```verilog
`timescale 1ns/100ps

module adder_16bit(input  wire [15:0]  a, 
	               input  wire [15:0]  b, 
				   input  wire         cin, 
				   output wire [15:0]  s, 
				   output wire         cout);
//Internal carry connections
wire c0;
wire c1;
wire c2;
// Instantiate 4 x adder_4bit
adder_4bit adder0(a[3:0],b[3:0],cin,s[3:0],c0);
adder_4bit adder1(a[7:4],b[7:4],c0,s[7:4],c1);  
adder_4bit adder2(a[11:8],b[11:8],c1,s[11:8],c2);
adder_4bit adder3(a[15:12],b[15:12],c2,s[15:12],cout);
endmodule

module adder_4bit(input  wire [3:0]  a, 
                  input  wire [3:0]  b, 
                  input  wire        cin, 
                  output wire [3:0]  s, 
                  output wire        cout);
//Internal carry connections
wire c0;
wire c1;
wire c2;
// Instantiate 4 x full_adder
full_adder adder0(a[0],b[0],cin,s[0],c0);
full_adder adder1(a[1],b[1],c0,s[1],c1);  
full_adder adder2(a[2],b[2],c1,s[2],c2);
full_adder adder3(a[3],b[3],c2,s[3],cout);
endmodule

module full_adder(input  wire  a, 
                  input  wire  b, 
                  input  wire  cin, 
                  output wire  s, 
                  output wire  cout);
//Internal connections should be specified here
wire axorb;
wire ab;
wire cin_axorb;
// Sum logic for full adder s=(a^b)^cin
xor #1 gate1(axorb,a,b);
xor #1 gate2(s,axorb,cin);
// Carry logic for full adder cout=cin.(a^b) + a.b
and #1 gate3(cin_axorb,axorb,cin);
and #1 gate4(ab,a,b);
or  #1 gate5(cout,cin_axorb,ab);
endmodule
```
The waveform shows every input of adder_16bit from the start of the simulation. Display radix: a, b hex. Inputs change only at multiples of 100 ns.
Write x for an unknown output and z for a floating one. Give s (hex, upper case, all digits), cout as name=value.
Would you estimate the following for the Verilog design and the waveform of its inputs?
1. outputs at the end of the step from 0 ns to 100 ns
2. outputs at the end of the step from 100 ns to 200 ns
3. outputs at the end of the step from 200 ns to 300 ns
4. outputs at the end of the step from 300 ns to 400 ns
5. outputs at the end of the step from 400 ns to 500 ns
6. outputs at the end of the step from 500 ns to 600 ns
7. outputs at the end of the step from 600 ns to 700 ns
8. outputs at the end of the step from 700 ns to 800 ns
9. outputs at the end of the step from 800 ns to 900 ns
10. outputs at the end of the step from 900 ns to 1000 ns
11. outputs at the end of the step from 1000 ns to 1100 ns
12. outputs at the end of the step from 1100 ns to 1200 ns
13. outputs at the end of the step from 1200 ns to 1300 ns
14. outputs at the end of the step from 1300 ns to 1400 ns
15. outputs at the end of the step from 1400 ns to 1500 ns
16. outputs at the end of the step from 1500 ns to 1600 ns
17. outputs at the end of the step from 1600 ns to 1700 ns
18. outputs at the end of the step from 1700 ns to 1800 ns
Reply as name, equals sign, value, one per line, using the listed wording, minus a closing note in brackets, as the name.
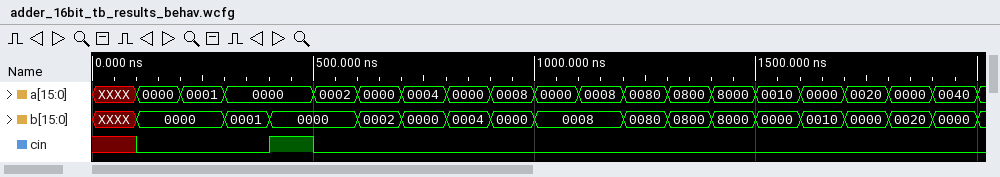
outputs at the end of the step from 0 ns to 100 ns = s=x, cout=x
outputs at the end of the step from 100 ns to 200 ns = s=0000, cout=0
outputs at the end of the step from 200 ns to 300 ns = s=0001, cout=0
outputs at the end of the step from 300 ns to 400 ns = s=0001, cout=0
outputs at the end of the step from 400 ns to 500 ns = s=0001, cout=0
outputs at the end of the step from 500 ns to 600 ns = s=0002, cout=0
outputs at the end of the step from 600 ns to 700 ns = s=0002, cout=0
outputs at the end of the step from 700 ns to 800 ns = s=0004, cout=0
outputs at the end of the step from 800 ns to 900 ns = s=0004, cout=0
outputs at the end of the step from 900 ns to 1000 ns = s=0008, cout=0
outputs at the end of the step from 1000 ns to 1100 ns = s=0008, cout=0
outputs at the end of the step from 1100 ns to 1200 ns = s=0010, cout=0
outputs at the end of the step from 1200 ns to 1300 ns = s=0100, cout=0
outputs at the end of the step from 1300 ns to 1400 ns = s=1000, cout=0
outputs at the end of the step from 1400 ns to 1500 ns = s=0000, cout=1
outputs at the end of the step from 1500 ns to 1600 ns = s=0010, cout=0
outputs at the end of the step from 1600 ns to 1700 ns = s=0010, cout=0
outputs at the end of the step from 1700 ns to 1800 ns = s=0020, cout=0
